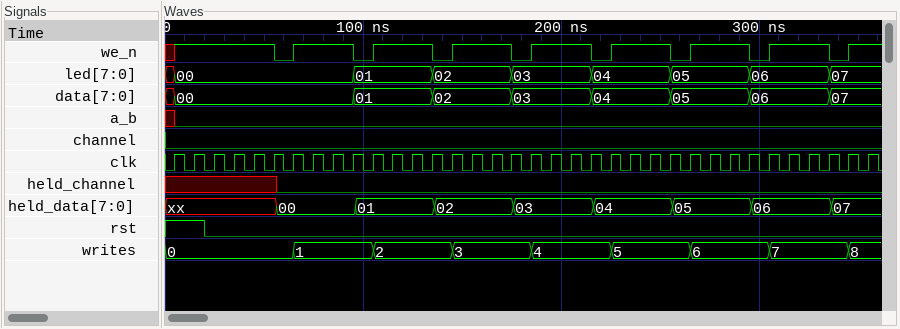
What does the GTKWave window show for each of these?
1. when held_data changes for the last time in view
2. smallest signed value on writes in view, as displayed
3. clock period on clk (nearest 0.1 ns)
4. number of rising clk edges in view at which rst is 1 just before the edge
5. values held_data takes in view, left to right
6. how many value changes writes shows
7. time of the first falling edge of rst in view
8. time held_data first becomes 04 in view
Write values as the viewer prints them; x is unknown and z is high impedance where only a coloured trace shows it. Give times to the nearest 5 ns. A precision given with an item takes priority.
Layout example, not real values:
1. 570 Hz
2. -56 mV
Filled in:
1. 335 ns
2. 0
3. 10 ns
4. 2
5. xx, 00, 01, 02, 03, 04, 05, 06, 07
6. 8
7. 20 ns
8. 215 ns
